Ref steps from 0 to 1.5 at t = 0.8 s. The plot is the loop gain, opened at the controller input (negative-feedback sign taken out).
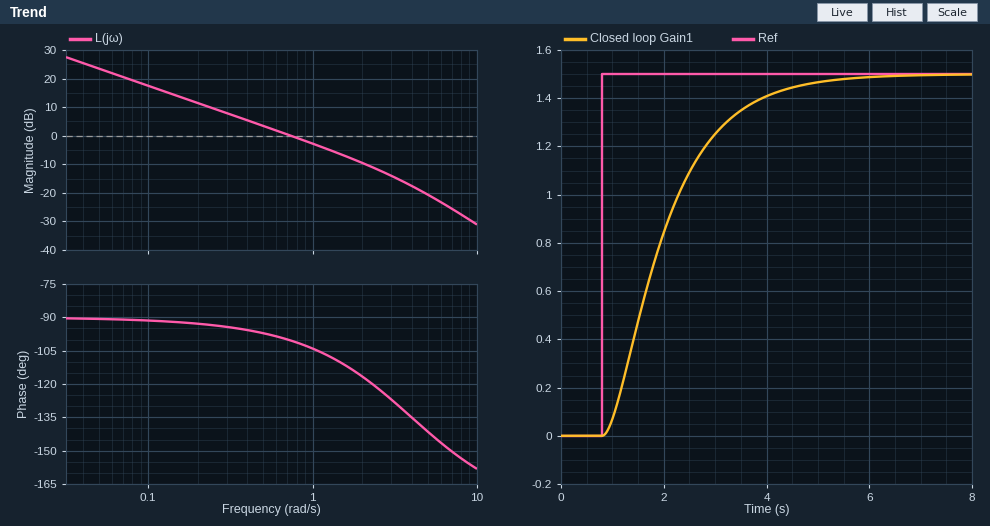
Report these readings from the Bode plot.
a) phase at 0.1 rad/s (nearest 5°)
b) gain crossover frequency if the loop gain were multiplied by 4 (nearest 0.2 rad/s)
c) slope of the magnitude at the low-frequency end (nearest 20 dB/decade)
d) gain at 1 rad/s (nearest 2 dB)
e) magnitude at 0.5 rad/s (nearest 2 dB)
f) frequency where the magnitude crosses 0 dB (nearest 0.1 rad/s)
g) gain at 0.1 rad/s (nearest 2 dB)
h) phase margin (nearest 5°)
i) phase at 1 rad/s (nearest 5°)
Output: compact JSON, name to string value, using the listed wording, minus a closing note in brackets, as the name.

{"phase at 0.1 rad/s": "-90°", "gain crossover frequency if the loop gain were multiplied by 4": "2.6 rad/s", "slope of the magnitude at the low-frequency end": "-20 dB/decade", "gain at 1 rad/s": "-2 dB", "magnitude at 0.5 rad/s": "4 dB", "frequency where the magnitude crosses 0 dB": "0.7 rad/s", "gain at 0.1 rad/s": "18 dB", "phase margin": "80°", "phase at 1 rad/s": "-105°"}
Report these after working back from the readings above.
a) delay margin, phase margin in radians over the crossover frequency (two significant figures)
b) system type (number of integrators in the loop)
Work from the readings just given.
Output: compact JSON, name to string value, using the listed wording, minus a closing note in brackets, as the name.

{"delay margin, phase margin in radians over the crossover frequency": "2.0 s", "system type": "1"}
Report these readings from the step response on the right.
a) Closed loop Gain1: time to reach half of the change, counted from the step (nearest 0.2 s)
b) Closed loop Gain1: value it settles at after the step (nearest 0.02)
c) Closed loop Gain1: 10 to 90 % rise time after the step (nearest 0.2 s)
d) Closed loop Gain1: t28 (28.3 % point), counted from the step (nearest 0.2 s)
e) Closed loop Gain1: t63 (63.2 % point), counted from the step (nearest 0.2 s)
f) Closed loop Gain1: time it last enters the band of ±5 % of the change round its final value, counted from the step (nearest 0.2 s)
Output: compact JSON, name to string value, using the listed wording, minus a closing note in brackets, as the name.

{"Closed loop Gain1: time to reach half of the change, counted from the step": "1.0 s", "Closed loop Gain1: value it settles at after the step": "1.50", "Closed loop Gain1: 10 to 90 % rise time after the step": "2.4 s", "Closed loop Gain1: t28 (28.3 % point), counted from the step": "0.6 s", "Closed loop Gain1: t63 (63.2 % point), counted from the step": "1.4 s", "Closed loop Gain1: time it last enters the band of ±5 % of the change round its final value, counted from the step": "3.4 s"}
